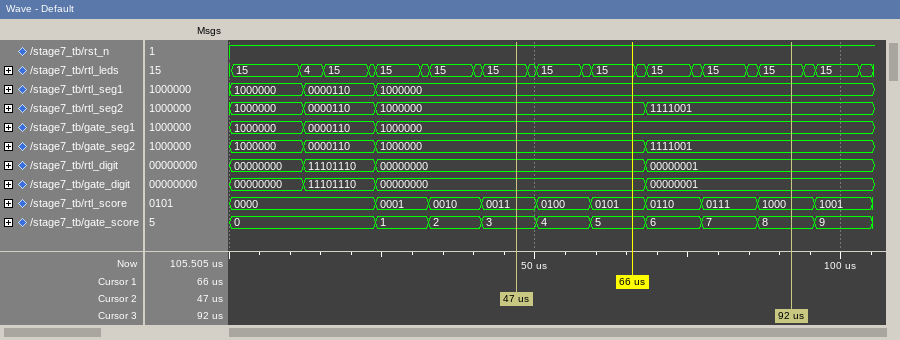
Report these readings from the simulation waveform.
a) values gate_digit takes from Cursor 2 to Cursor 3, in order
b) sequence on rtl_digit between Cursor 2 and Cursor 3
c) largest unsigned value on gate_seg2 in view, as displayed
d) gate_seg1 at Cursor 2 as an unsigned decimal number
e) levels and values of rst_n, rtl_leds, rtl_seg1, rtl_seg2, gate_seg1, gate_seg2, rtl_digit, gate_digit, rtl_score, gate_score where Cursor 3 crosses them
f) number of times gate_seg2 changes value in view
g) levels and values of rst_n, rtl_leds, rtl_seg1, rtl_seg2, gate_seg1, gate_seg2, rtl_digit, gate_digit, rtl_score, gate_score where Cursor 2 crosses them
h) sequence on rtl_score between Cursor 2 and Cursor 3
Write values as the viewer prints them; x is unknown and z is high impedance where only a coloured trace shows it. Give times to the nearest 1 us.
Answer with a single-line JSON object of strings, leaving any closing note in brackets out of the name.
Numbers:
{"values gate_digit takes from Cursor 2 to Cursor 3, in order": "00000000, 00000001", "sequence on rtl_digit between Cursor 2 and Cursor 3": "00000000, 00000001", "largest unsigned value on gate_seg2 in view, as displayed": "1111001", "gate_seg1 at Cursor 2 as an unsigned decimal number": "64", "levels and values of rst_n, rtl_leds, rtl_seg1, rtl_seg2, gate_seg1, gate_seg2, rtl_digit, gate_digit, rtl_score, gate_score where Cursor 3 crosses them": "rst_n=1, rtl_leds=15, rtl_seg1=1000000, rtl_seg2=1111001, gate_seg1=1000000, gate_seg2=1111001, rtl_digit=00000001, gate_digit=00000001, rtl_score=1000, gate_score=8", "number of times gate_seg2 changes value in view": "3", "levels and values of rst_n, rtl_leds, rtl_seg1, rtl_seg2, gate_seg1, gate_seg2, rtl_digit, gate_digit, rtl_score, gate_score where Cursor 2 crosses them": "rst_n=1, rtl_leds=15, rtl_seg1=1000000, rtl_seg2=1000000, gate_seg1=1000000, gate_seg2=1000000, rtl_digit=00000000, gate_digit=00000000, rtl_score=0011, gate_score=3", "sequence on rtl_score between Cursor 2 and Cursor 3": "0011, 0100, 0101, 0110, 0111, 1000"}
